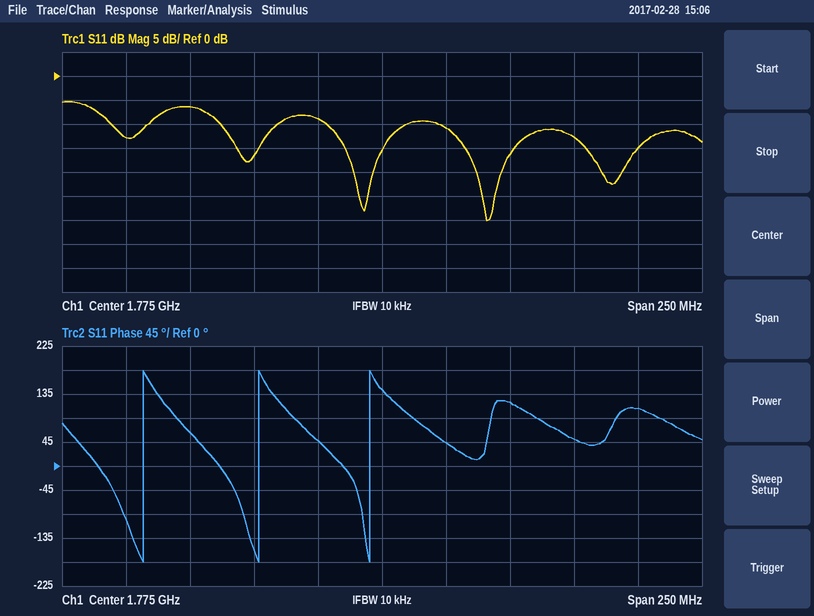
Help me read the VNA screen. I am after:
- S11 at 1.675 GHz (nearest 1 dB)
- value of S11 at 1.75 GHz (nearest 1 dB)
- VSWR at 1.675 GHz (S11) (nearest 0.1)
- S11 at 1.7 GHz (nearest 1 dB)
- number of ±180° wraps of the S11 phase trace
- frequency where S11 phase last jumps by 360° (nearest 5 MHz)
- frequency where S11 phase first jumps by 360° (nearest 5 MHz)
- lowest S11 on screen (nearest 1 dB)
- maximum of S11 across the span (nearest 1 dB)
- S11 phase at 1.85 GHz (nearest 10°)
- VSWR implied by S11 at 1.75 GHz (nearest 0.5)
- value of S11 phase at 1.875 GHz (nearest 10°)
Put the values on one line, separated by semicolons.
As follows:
-13 dB; -9 dB; 1.6; -6 dB; 3; 1.770 GHz; 1.680 GHz; -30 dB; -5 dB; 50°; 2.0; 110°
